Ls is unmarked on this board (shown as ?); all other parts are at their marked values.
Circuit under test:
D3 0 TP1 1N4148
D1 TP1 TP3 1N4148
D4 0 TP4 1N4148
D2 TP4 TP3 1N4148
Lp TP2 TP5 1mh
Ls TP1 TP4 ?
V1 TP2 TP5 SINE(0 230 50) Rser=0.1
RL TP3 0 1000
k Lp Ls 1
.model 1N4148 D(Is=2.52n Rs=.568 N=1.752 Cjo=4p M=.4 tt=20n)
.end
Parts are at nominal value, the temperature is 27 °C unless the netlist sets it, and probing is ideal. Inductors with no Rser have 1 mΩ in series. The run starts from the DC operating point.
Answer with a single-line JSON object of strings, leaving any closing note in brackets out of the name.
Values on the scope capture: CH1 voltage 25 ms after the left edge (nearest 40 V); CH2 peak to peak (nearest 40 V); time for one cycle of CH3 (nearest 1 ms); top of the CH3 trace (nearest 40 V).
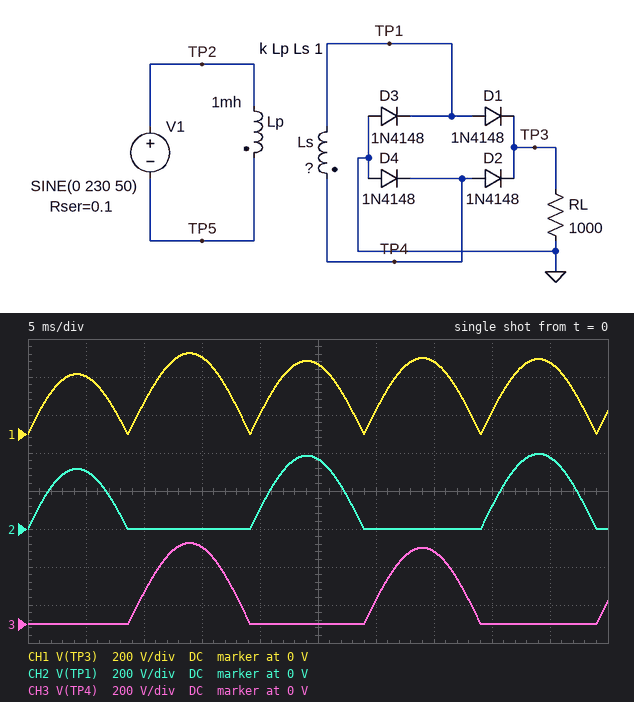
{"CH1 voltage 25 ms after the left edge": "360 V", "CH2 peak to peak": "400 V", "time for one cycle of CH3": "20 ms", "top of the CH3 trace": "440 V"}
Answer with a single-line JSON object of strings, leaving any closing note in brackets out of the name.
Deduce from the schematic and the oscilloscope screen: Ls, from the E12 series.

{"Ls, from the E12 series": "3.3 mH"}
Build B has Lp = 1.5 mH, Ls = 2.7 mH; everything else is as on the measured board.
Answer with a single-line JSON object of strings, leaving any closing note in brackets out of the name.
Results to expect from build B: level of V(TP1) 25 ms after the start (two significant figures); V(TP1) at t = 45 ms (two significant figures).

{"level of V(TP1) 25 ms after the start": "280 V", "V(TP1) at t = 45 ms": "290 V"}
